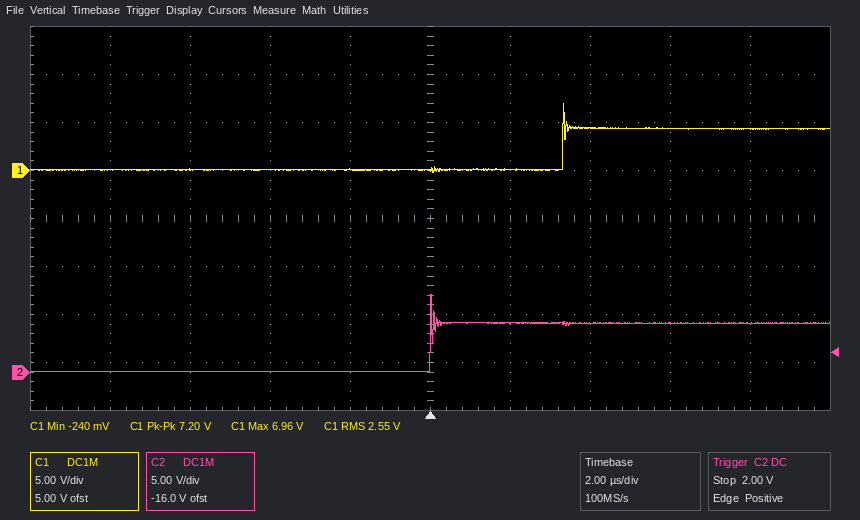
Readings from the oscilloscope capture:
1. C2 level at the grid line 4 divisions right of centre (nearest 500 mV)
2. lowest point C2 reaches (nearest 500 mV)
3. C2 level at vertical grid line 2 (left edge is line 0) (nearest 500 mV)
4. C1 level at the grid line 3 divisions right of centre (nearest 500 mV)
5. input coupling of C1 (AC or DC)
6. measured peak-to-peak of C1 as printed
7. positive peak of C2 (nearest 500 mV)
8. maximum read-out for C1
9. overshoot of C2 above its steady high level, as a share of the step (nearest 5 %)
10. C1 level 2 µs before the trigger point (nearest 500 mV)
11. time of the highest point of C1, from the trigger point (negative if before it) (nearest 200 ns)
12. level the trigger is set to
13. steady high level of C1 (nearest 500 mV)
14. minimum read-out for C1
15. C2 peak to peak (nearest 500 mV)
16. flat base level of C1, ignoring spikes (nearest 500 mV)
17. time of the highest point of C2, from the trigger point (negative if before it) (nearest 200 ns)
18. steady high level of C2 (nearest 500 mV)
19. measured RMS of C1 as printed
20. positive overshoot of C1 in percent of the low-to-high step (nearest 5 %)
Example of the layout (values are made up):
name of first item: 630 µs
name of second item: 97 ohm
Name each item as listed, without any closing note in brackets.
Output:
C2 level at the grid line 4 divisions right of centre: 5.0 V
lowest point C2 reaches: 0.0 V
C2 level at vertical grid line 2 (left edge is line 0): 0.0 V
C1 level at the grid line 3 divisions right of centre: 4.5 V
input coupling of C1: DC
measured peak-to-peak of C1 as printed: 7.20 V
positive peak of C2: 8.0 V
maximum read-out for C1: 6.96 V
overshoot of C2 above its steady high level, as a share of the step: 60 %
C1 level 2 µs before the trigger point: 0.0 V
time of the highest point of C1, from the trigger point (negative if before it): +3.4 µs
level the trigger is set to: 2.00 V
steady high level of C1: 4.5 V
minimum read-out for C1: -240 mV
C2 peak to peak: 8.0 V
flat base level of C1, ignoring spikes: 0.0 V
time of the highest point of C2, from the trigger point (negative if before it): 0.0 µs
steady high level of C2: 5.0 V
measured RMS of C1 as printed: 2.55 V
positive overshoot of C1 in percent of the low-to-high step: 60 %
